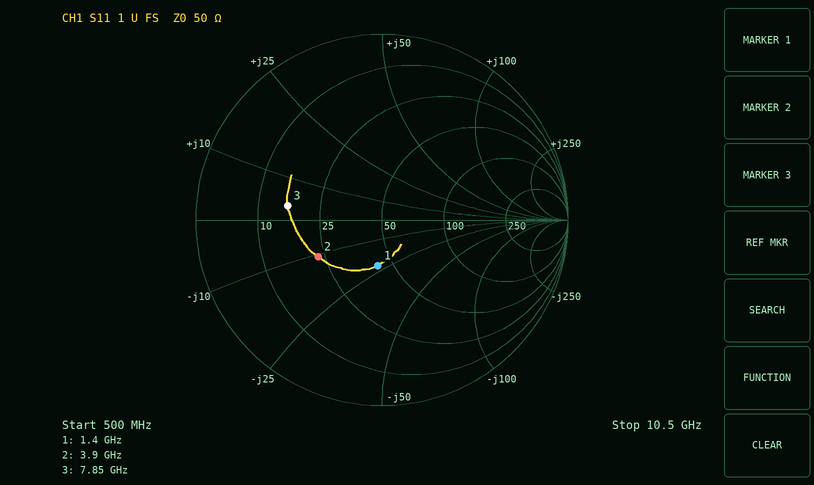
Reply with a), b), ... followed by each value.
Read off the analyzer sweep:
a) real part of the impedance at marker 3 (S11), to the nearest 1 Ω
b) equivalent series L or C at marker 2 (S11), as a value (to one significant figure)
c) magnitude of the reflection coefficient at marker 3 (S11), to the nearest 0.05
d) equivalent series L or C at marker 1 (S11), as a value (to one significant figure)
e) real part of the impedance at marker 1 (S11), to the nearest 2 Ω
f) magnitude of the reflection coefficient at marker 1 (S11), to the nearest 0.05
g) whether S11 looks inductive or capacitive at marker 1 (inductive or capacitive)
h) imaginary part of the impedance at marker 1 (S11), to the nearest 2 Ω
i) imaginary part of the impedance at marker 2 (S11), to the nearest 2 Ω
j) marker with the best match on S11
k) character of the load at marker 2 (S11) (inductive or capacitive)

a) 16 Ω
b) 4 pF
c) 0.50
d) 5 pF
e) 42 Ω
f) 0.25
g) capacitive
h) -22 Ω
i) -10 Ω
j) marker 1
k) capacitive
